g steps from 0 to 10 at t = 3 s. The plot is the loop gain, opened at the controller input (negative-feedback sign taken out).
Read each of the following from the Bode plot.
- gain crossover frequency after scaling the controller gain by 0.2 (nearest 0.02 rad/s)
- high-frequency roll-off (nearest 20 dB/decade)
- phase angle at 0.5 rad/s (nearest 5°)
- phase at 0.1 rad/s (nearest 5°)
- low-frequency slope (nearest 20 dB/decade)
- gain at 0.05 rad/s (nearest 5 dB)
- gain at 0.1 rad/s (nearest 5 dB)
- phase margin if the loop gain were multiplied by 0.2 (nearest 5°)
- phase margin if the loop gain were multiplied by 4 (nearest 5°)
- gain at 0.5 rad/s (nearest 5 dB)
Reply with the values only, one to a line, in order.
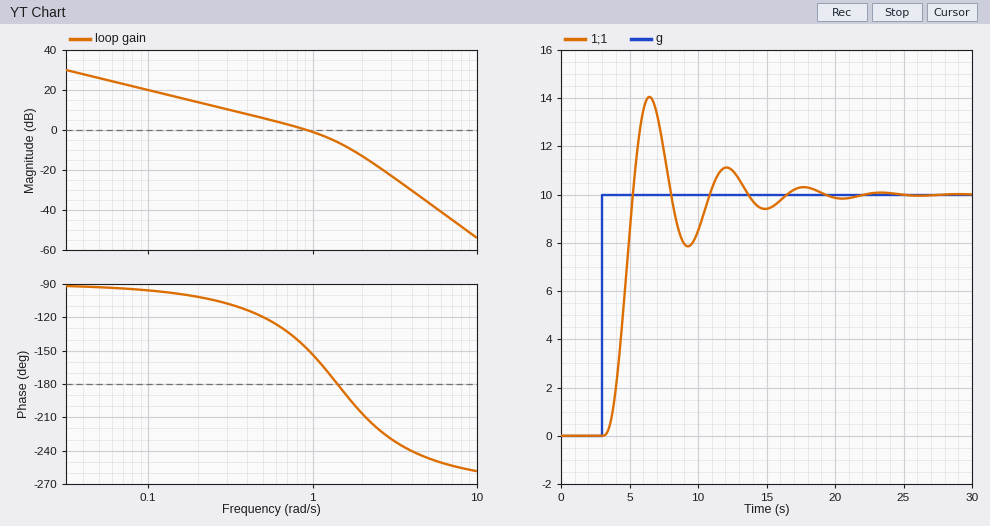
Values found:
0.20 rad/s
-60 dB/decade
-120°
-95°
-20 dB/decade
25 dB
20 dB
80°
-25°
5 dB
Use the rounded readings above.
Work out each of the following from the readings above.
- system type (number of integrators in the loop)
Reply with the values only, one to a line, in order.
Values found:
1
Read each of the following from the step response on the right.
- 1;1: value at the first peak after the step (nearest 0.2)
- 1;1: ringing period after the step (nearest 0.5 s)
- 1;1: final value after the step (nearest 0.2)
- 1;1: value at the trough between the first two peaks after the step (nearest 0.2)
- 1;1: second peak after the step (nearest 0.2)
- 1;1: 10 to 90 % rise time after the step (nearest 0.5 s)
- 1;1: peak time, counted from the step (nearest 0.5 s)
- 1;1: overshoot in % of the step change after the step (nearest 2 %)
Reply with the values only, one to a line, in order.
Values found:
14.0
5.5 s
10.0
7.8
11.2
1.5 s
3.5 s
40 %
